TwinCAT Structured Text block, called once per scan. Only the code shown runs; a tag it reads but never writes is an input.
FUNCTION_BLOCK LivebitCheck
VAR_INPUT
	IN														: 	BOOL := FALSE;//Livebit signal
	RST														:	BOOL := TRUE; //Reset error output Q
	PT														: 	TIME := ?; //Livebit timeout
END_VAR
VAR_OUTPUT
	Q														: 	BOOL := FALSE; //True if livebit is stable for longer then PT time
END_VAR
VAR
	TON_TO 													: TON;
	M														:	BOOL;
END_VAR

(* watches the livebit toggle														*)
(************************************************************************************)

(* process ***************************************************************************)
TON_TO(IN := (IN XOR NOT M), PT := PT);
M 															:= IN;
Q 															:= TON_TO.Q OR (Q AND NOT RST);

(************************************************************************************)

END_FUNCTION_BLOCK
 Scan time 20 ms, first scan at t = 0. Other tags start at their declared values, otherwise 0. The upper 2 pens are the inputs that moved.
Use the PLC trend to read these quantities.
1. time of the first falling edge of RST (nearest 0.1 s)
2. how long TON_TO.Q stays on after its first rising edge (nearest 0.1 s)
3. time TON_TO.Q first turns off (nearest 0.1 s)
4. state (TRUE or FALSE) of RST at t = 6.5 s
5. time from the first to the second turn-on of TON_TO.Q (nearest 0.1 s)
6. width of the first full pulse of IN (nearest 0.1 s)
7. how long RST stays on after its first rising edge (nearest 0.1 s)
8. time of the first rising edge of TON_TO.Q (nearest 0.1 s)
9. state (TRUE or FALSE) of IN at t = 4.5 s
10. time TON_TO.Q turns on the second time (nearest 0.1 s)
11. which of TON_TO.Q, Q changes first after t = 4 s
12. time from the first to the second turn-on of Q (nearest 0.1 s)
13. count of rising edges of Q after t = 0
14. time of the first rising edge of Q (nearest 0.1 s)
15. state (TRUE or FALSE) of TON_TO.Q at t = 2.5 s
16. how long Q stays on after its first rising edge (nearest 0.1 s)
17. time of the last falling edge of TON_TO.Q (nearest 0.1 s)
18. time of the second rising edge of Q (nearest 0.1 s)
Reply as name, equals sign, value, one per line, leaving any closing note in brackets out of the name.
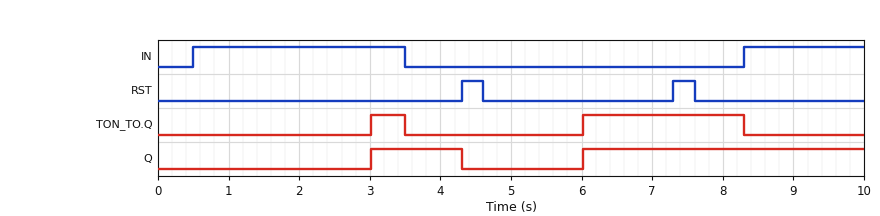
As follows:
time of the first falling edge of RST = 4.6 s
how long TON_TO.Q stays on after its first rising edge = 0.5 s
time TON_TO.Q first turns off = 3.5 s
state (TRUE or FALSE) of RST at t = 6.5 s = FALSE
time from the first to the second turn-on of TON_TO.Q = 3.0 s
width of the first full pulse of IN = 3.0 s
how long RST stays on after its first rising edge = 0.3 s
time of the first rising edge of TON_TO.Q = 3.0 s
state (TRUE or FALSE) of IN at t = 4.5 s = FALSE
time TON_TO.Q turns on the second time = 6.0 s
which of TON_TO.Q, Q changes first after t = 4 s = Q
time from the first to the second turn-on of Q = 3.0 s
count of rising edges of Q after t = 0 = 2
time of the first rising edge of Q = 3.0 s
state (TRUE or FALSE) of TON_TO.Q at t = 2.5 s = FALSE
how long Q stays on after its first rising edge = 1.3 s
time of the last falling edge of TON_TO.Q = 8.3 s
time of the second rising edge of Q = 6.0 s
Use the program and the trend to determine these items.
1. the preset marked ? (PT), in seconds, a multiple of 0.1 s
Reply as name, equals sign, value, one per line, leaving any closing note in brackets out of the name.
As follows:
the preset marked ? (PT), in seconds, a multiple of 0.1 s = 2.5 s
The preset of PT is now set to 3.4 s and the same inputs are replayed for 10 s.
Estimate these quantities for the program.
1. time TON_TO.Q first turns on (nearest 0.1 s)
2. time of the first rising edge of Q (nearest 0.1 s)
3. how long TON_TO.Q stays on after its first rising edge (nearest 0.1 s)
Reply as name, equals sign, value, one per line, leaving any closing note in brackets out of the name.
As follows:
time TON_TO.Q first turns on = 6.9 s
time of the first rising edge of Q = 6.9 s
how long TON_TO.Q stays on after its first rising edge = 1.4 s
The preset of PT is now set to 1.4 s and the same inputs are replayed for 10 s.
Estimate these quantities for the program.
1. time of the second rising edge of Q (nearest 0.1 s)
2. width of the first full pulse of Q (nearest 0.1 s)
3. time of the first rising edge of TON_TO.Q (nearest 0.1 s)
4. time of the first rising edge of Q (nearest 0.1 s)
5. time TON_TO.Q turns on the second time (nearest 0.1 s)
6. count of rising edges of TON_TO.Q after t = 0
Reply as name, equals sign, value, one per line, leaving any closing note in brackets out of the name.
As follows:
time of the second rising edge of Q = 4.9 s
width of the first full pulse of Q = 2.4 s
time of the first rising edge of TON_TO.Q = 1.9 s
time of the first rising edge of Q = 1.9 s
time TON_TO.Q turns on the second time = 4.9 s
count of rising edges of TON_TO.Q after t = 0 = 3
